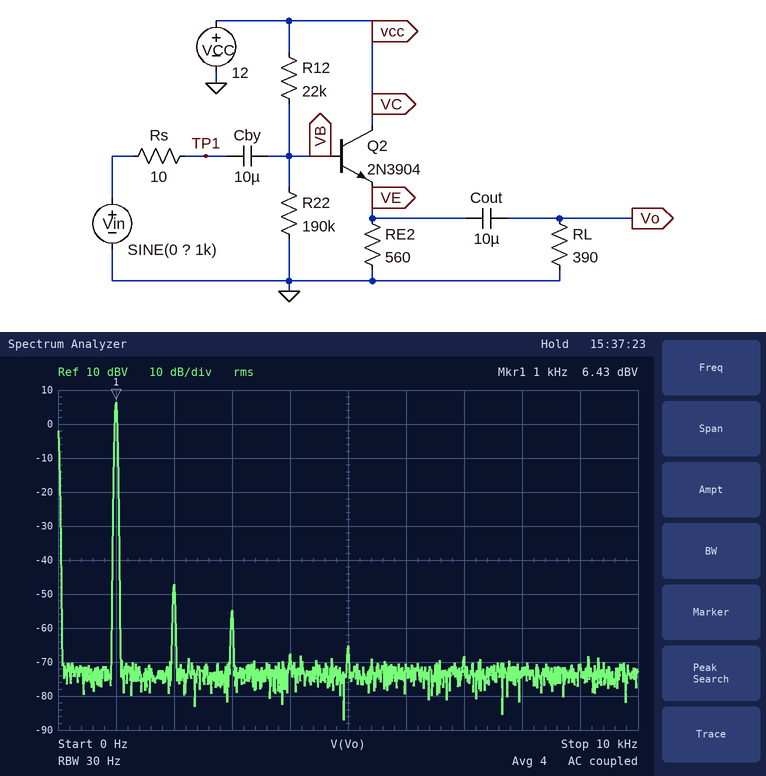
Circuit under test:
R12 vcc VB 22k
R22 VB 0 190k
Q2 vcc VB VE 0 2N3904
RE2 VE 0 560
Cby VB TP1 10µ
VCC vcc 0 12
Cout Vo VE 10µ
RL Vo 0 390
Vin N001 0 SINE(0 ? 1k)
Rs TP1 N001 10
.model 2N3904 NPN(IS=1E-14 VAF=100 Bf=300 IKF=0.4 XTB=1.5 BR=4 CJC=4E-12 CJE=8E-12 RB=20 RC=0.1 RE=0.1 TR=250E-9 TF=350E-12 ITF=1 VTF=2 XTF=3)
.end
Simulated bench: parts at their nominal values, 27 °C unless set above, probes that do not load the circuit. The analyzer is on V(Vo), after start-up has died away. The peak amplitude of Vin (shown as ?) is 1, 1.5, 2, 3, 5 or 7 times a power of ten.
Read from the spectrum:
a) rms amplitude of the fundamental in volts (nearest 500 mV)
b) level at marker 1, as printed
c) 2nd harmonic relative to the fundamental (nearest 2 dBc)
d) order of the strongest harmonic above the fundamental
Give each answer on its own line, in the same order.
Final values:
2.0 V
6.43 dBV
-54 dBc
2
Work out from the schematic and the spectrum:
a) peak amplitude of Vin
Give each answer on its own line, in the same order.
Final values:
3 V
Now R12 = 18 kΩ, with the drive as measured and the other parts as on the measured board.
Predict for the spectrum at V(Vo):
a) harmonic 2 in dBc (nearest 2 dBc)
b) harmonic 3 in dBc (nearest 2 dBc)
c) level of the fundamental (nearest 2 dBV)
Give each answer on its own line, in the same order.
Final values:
-56 dBc
-58 dBc
6 dBV
